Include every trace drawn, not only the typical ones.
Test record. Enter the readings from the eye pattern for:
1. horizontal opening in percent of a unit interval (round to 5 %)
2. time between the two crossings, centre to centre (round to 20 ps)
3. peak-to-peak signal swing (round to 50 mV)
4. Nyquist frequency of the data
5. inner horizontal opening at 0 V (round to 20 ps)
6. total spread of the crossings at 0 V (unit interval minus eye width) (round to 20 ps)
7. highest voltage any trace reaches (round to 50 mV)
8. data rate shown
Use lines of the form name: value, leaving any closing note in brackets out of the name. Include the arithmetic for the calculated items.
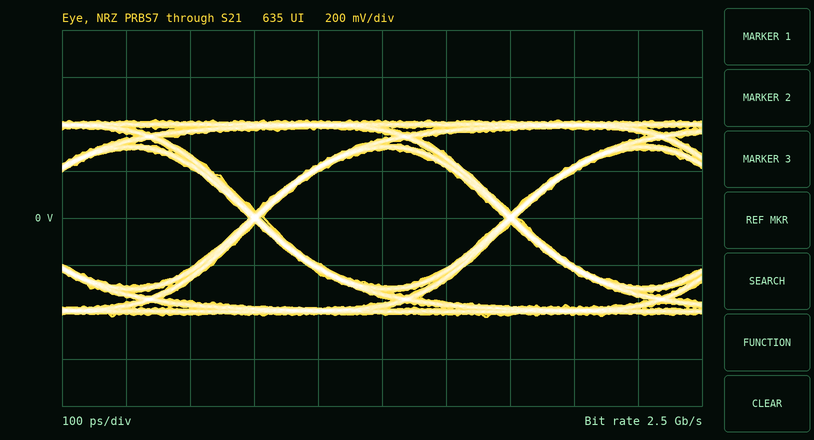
horizontal opening in percent of a unit interval: 380 ps / 400 ps ≈ 95 %
time between the two crossings, centre to centre: 400 ps
peak-to-peak signal swing: 850 mV
Nyquist frequency of the data: 1.25 GHz
inner horizontal opening at 0 V: 380 ps
total spread of the crossings at 0 V (unit interval minus eye width): 20 ps
highest voltage any trace reaches: 400 mV
data rate shown: 2.5 Gb/s
